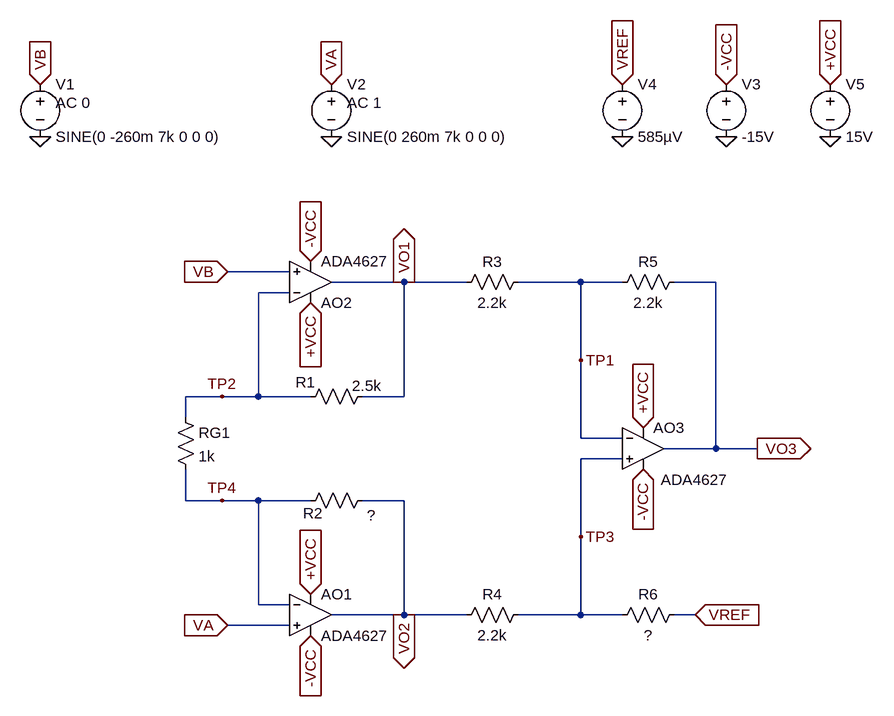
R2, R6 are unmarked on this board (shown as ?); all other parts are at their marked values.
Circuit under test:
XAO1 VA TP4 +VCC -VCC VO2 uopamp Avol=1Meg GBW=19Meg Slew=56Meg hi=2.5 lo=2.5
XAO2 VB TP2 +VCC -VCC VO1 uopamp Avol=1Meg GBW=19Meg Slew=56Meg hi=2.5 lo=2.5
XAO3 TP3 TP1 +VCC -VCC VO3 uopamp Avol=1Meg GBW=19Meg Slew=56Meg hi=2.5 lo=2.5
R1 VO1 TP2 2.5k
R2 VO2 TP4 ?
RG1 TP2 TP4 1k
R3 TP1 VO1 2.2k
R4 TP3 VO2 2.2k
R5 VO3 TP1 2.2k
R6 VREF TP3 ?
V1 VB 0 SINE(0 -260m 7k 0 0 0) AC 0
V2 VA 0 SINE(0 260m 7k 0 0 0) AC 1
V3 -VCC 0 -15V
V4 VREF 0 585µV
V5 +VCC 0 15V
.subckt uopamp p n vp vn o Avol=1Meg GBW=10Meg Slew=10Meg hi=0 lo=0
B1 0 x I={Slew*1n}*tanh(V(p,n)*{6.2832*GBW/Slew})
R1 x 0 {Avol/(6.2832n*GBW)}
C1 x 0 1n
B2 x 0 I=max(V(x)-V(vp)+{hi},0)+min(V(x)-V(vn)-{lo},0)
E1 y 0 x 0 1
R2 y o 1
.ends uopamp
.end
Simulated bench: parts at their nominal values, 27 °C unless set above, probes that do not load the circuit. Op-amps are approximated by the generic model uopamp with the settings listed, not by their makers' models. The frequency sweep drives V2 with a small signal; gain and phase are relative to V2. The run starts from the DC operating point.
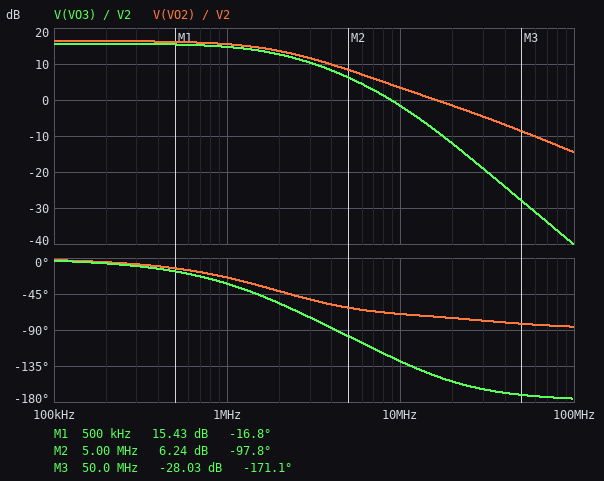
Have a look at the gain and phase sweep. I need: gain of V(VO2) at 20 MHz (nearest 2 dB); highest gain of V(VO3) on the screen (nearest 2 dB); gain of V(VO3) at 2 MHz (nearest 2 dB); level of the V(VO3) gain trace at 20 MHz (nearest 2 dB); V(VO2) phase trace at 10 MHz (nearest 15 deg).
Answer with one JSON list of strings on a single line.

["-2 dB", "16 dB", "12 dB", "-12 dB", "-75 deg"]
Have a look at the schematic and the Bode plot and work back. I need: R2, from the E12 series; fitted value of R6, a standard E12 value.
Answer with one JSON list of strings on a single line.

["5.6 kΩ", "820 Ω"]
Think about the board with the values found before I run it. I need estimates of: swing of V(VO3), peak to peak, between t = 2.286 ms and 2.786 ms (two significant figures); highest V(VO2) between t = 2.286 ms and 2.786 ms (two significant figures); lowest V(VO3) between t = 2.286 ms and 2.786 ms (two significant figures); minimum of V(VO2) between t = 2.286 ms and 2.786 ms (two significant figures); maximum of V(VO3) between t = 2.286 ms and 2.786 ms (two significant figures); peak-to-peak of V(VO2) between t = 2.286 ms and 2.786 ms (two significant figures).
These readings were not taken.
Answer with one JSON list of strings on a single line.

["6.6 V", "3.2 V", "-3.3 V", "-3.2 V", "3.3 V", "6.3 V"]
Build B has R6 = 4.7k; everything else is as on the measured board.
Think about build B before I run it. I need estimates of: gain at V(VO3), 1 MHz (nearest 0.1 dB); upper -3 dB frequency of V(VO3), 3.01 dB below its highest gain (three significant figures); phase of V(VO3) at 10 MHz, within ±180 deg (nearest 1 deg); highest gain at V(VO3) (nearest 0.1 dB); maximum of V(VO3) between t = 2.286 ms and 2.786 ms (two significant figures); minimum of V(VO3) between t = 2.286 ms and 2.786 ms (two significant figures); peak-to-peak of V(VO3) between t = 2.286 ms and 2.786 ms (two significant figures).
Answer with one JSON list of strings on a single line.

["20.3 dB", "2.00 MHz", "-123 deg", "21.2 dB", "5.9 V", "-5.9 V", "12 V"]
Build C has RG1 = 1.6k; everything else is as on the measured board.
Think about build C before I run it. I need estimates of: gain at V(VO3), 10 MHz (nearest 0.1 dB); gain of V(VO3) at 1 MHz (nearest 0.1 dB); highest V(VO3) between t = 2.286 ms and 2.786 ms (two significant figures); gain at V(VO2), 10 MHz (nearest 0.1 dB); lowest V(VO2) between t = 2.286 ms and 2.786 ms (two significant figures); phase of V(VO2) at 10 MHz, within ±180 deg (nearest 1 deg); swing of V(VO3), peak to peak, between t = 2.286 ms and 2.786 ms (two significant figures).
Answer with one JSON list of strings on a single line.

["-2.0 dB", "11.6 dB", "2.2 V", "3.3 dB", "-2.1 V", "-65 deg", "4.4 V"]
